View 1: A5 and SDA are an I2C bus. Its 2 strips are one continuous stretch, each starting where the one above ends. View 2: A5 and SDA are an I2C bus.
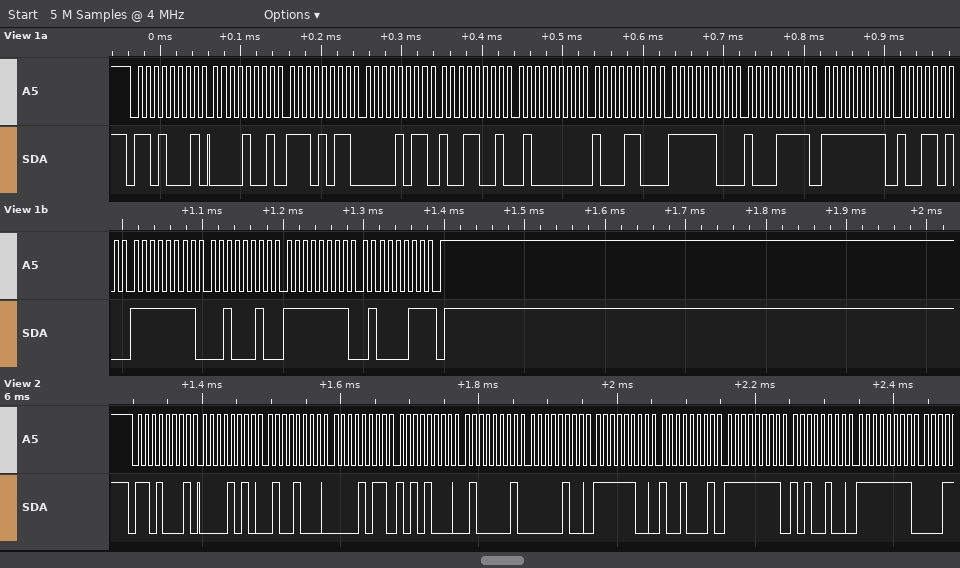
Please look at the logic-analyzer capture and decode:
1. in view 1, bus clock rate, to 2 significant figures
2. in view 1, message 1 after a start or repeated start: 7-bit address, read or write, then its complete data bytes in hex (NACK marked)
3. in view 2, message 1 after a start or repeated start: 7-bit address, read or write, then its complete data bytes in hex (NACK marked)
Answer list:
100 kHz
0x68 read: 09 EB 0B 99 40 8C FC 8F FF 9A FF 22 FF 43 NACK
0x68 read: 0A 48 0B A8 41 04 FC 91 FF A4 FF
